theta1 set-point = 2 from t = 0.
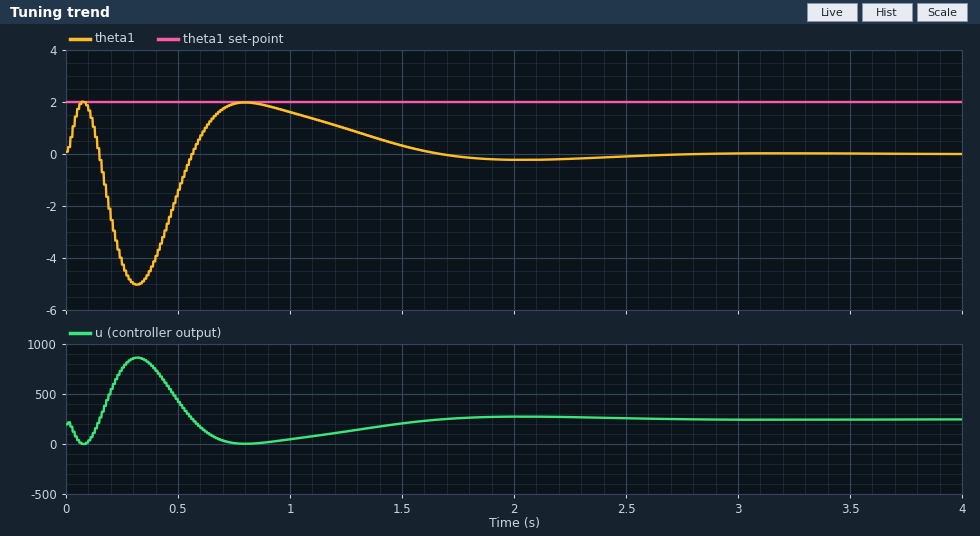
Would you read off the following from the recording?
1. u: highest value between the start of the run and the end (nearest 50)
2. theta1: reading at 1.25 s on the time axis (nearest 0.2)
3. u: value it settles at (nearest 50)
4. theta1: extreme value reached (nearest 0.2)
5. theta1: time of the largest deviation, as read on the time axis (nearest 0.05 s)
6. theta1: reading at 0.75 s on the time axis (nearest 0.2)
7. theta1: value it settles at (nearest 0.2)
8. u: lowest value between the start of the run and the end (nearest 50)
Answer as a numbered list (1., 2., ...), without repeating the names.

1. 850
2. 1.0
3. 250
4. -5.0
5. 0.30 s
6. 2.0
7. 0.0
8. 0
